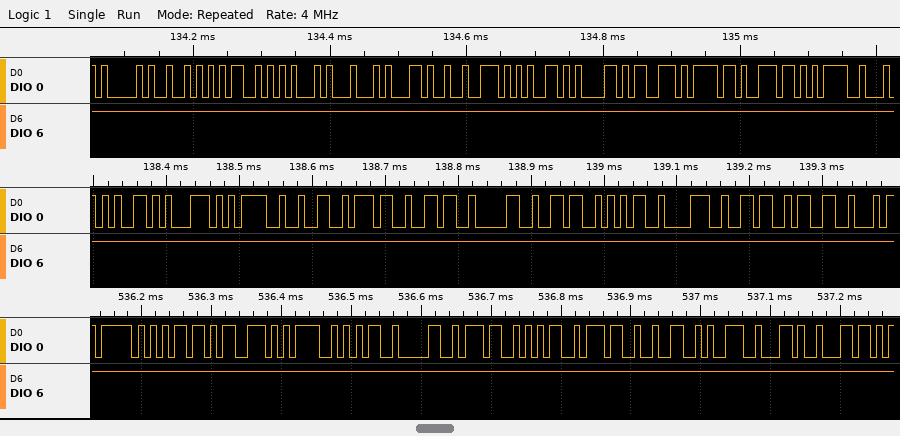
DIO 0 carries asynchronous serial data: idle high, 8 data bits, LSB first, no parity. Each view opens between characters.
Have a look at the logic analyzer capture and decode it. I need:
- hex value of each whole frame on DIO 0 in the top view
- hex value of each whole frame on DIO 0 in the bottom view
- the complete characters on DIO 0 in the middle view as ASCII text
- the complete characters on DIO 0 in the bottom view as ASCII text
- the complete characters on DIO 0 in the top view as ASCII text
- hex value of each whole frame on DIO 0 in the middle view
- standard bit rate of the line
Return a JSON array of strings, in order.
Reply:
["41, 52, 4D, 45, 44, 2C, 72, 65, 61, 73, 6F, 6E, 3D", "5F, 6D, 73, 3D, 35, 30, 37, 35, 37, 32, 39, 2C, 6C", "\"eq=276065863\"", "\"_ms=5075729,l\"", "\"ARMED,reason=\"", "65, 71, 3D, 32, 37, 36, 30, 36, 35, 38, 36, 33", "115200 baud"]
